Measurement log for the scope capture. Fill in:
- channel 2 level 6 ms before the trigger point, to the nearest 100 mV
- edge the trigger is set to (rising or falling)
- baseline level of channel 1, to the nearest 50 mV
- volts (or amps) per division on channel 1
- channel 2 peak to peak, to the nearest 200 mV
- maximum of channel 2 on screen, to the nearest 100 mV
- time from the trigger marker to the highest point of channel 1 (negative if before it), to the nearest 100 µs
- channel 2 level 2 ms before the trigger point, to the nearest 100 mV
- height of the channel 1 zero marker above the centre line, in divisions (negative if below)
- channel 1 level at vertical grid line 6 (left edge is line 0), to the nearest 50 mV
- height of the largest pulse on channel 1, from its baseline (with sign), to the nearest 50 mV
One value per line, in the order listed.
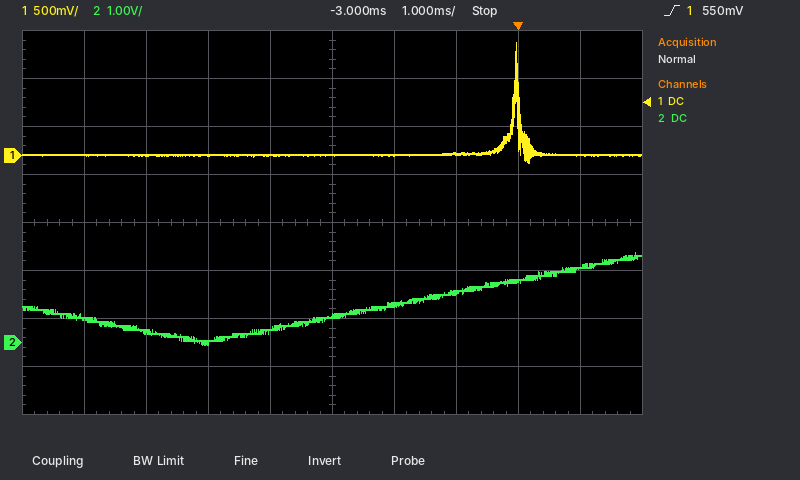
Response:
200 mV
rising
0 mV
500 mV
2.0 V
1.9 V
0.0 ms
800 mV
+1.4 div
0 mV
+1.15 V
